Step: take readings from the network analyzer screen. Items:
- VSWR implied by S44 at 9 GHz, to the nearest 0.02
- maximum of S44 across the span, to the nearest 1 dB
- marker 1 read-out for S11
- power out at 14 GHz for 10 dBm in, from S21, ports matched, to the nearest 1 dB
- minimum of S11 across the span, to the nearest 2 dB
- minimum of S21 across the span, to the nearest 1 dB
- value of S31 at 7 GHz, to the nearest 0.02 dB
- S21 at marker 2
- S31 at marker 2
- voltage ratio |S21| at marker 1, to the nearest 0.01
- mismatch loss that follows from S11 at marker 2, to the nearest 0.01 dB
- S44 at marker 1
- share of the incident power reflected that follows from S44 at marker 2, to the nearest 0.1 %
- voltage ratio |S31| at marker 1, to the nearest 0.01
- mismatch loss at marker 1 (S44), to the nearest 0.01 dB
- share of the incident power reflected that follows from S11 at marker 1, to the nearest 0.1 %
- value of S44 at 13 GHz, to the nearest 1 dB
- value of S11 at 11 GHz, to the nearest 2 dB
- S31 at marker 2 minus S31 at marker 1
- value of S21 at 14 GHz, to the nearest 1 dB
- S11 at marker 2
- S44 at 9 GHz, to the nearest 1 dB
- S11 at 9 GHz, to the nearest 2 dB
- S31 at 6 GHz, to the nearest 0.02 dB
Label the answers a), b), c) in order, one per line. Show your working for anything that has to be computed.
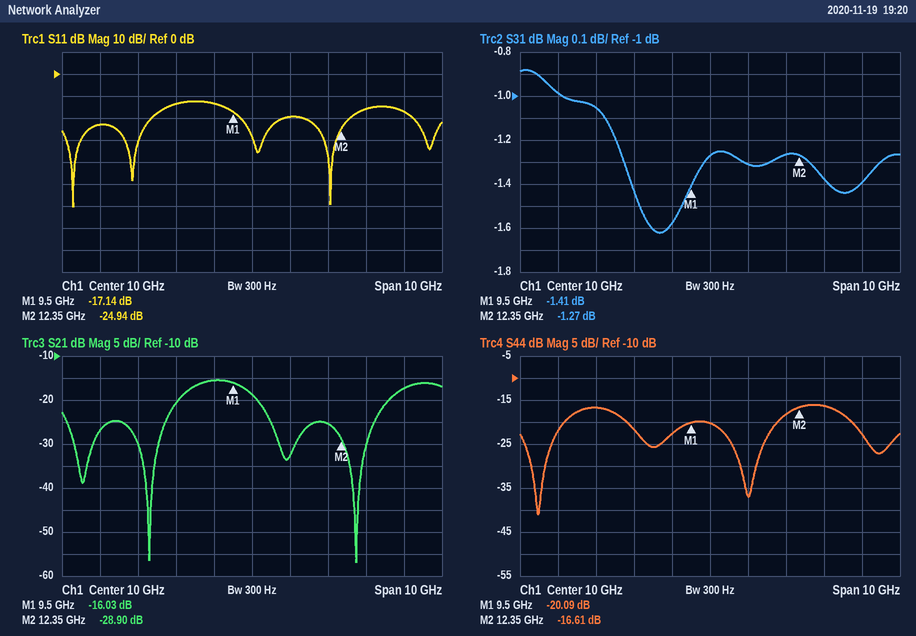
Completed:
a) |Γ| = 10^(-23/20) = 0.0708; VSWR = (1 + 0.0708)/(1 − 0.0708) ≈ 1.15, so 1.16 to the nearest 0.02
b) -16 dB
c) -17.14 dB
d) 10 dBm + (-17 dB) = -7 dBm
e) -60 dB
f) -57 dB
g) -1.06 dB
h) -28.90 dB
i) -1.27 dB
j) 10^(-16.03/20) ≈ 0.16
k) −10 log10(1 − 10^(-24.94/10)) ≈ 0.01 dB
l) -20.09 dB
m) 10^(-16.61/10) ≈ 2.2 %
n) 10^(-1.41/20) ≈ 0.85
o) −10 log10(1 − 10^(-20.09/10)) ≈ 0.04 dB
p) 10^(-17.14/10) ≈ 1.9 %
q) -16 dB
r) -20 dB
s) -1.27 − (-1.41) = 0.14 dB
t) -17 dB
u) -24.94 dB
v) -23 dB
w) -14 dB
x) -0.98 dB
